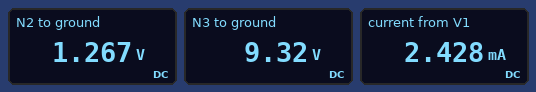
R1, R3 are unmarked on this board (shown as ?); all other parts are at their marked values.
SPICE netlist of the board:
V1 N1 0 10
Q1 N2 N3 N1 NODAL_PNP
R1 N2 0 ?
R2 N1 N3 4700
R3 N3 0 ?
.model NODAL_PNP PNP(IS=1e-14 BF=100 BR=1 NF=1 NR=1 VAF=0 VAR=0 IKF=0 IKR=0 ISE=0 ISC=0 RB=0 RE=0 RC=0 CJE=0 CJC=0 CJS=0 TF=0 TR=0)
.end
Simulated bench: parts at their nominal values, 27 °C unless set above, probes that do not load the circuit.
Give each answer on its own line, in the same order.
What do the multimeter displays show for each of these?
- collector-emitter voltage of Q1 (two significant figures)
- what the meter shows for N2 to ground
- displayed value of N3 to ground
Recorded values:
-8.7 V
1.267 V
9.32 V
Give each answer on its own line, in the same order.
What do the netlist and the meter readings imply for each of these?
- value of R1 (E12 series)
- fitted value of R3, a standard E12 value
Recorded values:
560 Ω
56 kΩ
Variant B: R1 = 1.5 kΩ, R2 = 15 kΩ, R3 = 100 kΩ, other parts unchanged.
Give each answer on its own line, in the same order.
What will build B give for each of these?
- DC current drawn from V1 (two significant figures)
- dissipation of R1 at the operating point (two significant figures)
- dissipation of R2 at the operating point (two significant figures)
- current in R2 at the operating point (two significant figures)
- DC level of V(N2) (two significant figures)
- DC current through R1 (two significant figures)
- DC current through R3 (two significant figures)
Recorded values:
4.8 mA
33 mW
32 µW
46 µA
7.0 V
4.7 mA
93 µA
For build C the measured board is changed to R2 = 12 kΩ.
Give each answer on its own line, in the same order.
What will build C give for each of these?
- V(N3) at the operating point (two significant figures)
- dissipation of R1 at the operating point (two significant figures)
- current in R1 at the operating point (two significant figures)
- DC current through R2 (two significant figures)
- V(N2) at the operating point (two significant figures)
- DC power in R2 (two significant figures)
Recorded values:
9.3 V
63 mW
11 mA
60 µA
5.9 V
43 µW
